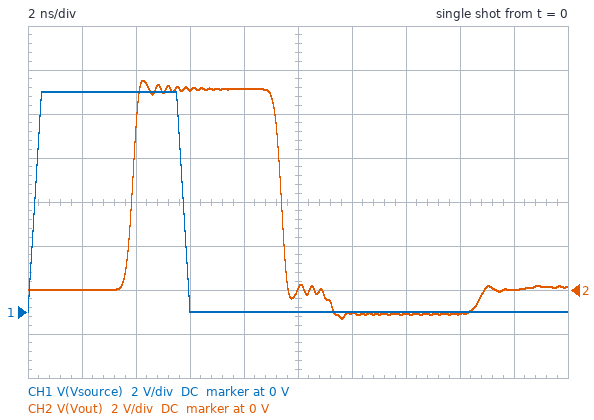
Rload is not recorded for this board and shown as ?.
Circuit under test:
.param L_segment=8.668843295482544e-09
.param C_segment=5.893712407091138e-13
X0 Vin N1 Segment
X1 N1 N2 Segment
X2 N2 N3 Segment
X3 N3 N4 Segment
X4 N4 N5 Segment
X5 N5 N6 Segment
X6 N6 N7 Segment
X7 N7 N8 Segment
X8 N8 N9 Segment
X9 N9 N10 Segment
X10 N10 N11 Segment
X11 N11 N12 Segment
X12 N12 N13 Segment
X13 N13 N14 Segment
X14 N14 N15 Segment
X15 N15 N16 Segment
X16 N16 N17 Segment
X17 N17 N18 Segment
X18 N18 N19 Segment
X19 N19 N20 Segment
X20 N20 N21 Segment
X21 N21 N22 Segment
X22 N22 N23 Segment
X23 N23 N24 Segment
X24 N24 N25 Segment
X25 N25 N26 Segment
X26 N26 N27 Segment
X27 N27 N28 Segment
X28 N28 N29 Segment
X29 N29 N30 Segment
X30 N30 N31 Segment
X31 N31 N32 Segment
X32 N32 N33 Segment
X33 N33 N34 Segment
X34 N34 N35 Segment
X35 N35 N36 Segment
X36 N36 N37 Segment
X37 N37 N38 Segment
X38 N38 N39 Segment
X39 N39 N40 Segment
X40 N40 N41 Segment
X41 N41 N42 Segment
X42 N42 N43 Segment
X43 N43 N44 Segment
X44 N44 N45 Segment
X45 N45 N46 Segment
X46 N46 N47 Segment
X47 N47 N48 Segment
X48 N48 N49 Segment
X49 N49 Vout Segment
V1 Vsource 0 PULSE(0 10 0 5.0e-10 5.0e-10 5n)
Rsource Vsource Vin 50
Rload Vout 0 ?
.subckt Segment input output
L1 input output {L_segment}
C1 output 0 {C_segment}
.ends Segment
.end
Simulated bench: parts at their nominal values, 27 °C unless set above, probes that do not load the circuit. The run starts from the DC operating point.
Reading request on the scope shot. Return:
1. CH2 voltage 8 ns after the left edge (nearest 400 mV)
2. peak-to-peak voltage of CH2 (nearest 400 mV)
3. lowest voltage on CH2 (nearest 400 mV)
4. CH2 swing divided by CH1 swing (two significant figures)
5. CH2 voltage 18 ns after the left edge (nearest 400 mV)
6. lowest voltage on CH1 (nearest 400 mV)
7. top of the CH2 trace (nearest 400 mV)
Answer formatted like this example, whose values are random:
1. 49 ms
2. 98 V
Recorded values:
1. 9.2 V
2. 10.8 V
3. -1.2 V
4. 1.1
5. 0 V
6. 0 V
7. 9.6 V
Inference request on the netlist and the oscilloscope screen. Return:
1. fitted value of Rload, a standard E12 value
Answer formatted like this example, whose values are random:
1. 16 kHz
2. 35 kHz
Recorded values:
1. 220 Ω
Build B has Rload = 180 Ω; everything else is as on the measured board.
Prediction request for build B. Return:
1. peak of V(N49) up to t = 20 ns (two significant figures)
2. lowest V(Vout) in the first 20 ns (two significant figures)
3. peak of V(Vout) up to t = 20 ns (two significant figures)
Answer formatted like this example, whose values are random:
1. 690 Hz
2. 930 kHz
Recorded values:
1. 8.7 V
2. -840 mV
3. 8.8 V
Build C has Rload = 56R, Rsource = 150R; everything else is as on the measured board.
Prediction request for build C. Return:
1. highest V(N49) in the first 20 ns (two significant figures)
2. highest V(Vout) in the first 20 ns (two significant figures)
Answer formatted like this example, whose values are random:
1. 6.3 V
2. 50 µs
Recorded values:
1. 3.1 V
2. 2.9 V
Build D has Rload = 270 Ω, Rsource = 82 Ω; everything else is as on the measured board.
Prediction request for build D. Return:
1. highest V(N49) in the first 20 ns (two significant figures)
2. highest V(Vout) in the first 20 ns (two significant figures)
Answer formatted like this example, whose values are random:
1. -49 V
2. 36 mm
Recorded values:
1. 8.5 V
2. 8.6 V
